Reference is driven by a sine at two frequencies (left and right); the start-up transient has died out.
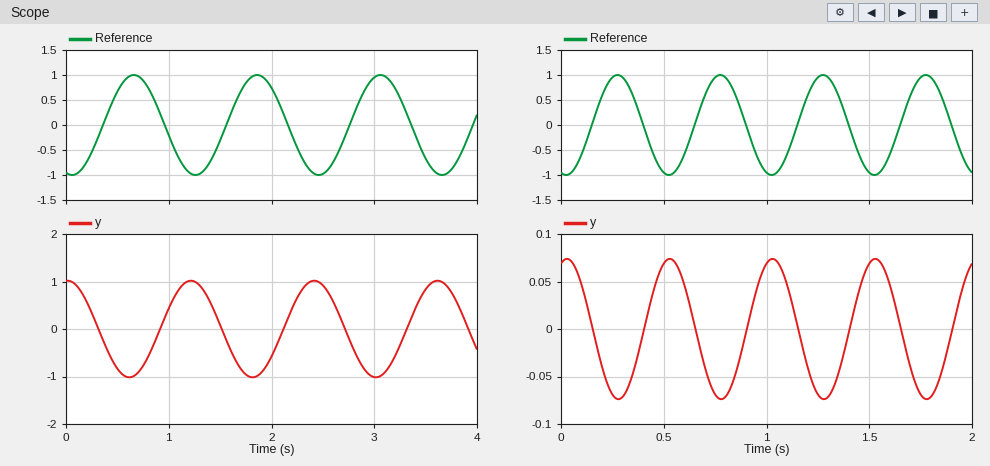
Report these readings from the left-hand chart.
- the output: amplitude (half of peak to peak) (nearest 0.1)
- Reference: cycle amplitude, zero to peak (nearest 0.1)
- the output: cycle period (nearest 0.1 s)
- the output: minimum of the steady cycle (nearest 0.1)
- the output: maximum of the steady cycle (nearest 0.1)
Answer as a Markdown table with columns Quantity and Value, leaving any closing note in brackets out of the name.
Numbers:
| Quantity | Value |
|---|---|
| the output: amplitude (half of peak to peak) | 1.0 |
| Reference: cycle amplitude, zero to peak | 1.0 |
| the output: cycle period | 1.2 s |
| the output: minimum of the steady cycle | -1.0 |
| the output: maximum of the steady cycle | 1.0 |
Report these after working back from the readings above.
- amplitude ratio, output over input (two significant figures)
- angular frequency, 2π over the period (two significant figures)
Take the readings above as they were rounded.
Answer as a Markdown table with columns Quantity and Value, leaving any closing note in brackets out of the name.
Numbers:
| Quantity | Value |
|---|---|
| amplitude ratio, output over input | 1.0 |
| angular frequency, 2π over the period | 5.2 rad/s |
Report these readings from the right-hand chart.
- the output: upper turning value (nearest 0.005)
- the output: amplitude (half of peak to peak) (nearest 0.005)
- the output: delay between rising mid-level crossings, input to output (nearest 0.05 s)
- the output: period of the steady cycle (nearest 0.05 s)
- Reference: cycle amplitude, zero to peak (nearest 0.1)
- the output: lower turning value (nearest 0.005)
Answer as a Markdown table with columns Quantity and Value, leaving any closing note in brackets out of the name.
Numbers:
| Quantity | Value |
|---|---|
| the output: upper turning value | 0.075 |
| the output: amplitude (half of peak to peak) | 0.075 |
| the output: delay between rising mid-level crossings, input to output | 0.25 s |
| the output: period of the steady cycle | 0.50 s |
| Reference: cycle amplitude, zero to peak | 1.0 |
| the output: lower turning value | -0.075 |
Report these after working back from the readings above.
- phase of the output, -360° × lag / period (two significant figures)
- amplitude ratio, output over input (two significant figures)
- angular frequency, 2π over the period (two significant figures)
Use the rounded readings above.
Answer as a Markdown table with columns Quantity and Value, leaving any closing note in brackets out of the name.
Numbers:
| Quantity | Value |
|---|---|
| phase of the output, -360° × lag / period | -180° |
| amplitude ratio, output over input | 0.075 |
| angular frequency, 2π over the period | 13 rad/s |
